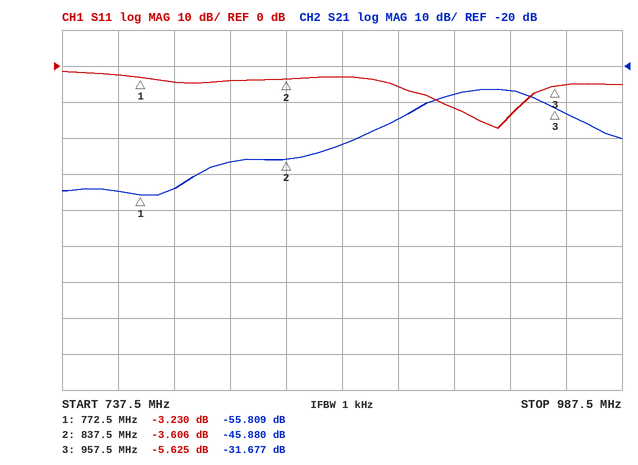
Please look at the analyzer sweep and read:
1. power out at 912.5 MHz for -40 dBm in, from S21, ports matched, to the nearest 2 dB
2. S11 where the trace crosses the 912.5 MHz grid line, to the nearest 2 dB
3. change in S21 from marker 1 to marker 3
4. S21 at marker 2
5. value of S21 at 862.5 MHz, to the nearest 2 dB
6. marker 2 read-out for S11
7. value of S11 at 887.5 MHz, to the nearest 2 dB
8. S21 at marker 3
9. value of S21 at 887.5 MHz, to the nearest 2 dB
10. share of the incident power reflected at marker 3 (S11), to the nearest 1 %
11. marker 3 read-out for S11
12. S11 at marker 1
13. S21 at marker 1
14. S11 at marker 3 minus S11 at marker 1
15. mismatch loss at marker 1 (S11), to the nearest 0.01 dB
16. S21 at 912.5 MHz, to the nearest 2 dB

-68 dBm
-12 dB
24.132 dB
-45.880 dB
-42 dB
-3.606 dB
-6 dB
-31.677 dB
-34 dB
27 %
-5.625 dB
-3.230 dB
-55.809 dB
-2.395 dB
2.80 dB
-28 dB
